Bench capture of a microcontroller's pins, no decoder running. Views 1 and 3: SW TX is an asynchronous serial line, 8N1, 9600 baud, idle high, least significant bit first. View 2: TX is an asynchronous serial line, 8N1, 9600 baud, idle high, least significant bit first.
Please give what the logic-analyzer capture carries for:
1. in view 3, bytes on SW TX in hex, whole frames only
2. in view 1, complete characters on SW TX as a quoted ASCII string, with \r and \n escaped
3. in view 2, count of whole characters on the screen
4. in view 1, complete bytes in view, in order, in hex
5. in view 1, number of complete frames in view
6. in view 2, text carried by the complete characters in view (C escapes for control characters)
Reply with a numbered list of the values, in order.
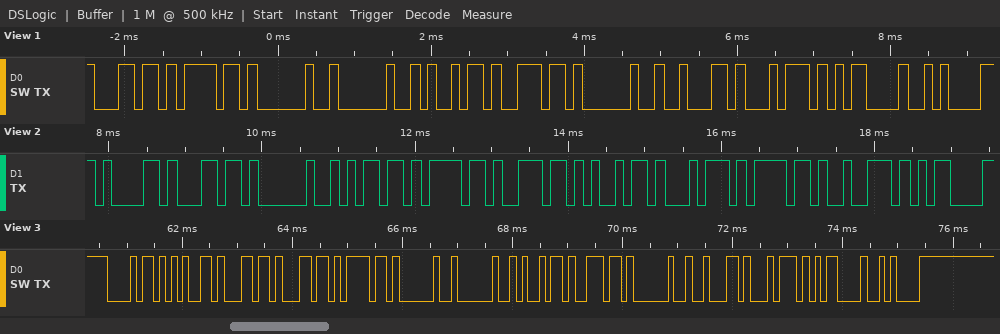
1. 0x68 0x65 0x6C 0x6C 0x6F 0x20 0x20 0x69 0x6E 0x20 0x62 0x74 0x0D 0x0A
2. "lo  in bt\r\n"
3. 11
4. 0x6C 0x6F 0x20 0x20 0x69 0x6E 0x20 0x62 0x74 0x0D 0x0A
5. 11
6. "al monitor\r"
